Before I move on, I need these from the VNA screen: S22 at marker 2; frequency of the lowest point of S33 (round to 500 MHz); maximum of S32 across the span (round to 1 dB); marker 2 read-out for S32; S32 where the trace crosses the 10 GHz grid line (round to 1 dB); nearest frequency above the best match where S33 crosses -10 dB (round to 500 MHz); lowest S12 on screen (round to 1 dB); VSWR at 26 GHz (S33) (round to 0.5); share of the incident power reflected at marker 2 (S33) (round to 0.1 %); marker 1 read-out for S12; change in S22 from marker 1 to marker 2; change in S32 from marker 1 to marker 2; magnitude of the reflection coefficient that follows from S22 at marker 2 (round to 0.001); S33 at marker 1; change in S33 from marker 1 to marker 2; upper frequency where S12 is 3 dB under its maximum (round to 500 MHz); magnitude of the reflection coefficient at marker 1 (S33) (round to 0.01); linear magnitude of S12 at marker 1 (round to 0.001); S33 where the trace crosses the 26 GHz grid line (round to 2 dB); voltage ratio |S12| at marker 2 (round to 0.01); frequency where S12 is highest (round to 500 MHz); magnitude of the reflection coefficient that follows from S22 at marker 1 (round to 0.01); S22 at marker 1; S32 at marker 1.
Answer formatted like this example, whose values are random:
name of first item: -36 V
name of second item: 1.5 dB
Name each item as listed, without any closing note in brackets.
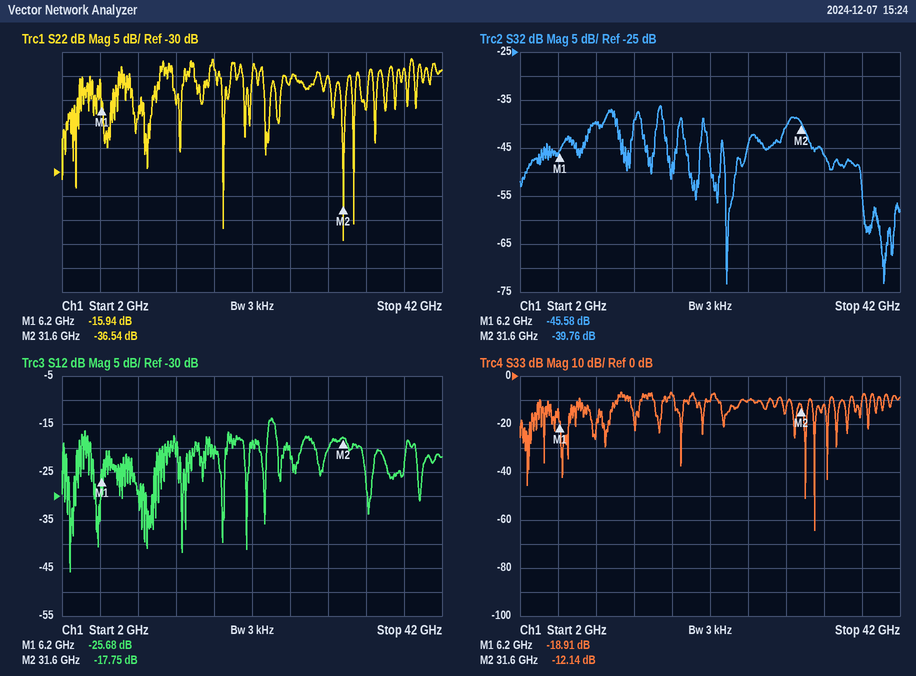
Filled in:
S22 at marker 2: -36.54 dB
frequency of the lowest point of S33: 33.0 GHz
maximum of S32 across the span: -36 dB
marker 2 read-out for S32: -39.76 dB
S32 where the trace crosses the 10 GHz grid line: -40 dB
nearest frequency above the best match where S33 crosses -10 dB: 34.5 GHz
lowest S12 on screen: -46 dB
VSWR at 26 GHz (S33): 2.0
share of the incident power reflected at marker 2 (S33): 6.1 %
marker 1 read-out for S12: -25.68 dB
change in S22 from marker 1 to marker 2: -20.60 dB
change in S32 from marker 1 to marker 2: 5.82 dB
magnitude of the reflection coefficient that follows from S22 at marker 2: 0.015
S33 at marker 1: -18.91 dB
change in S33 from marker 1 to marker 2: 6.77 dB
upper frequency where S12 is 3 dB under its maximum: 24.5 GHz
magnitude of the reflection coefficient at marker 1 (S33): 0.11
linear magnitude of S12 at marker 1: 0.052
S33 where the trace crosses the 26 GHz grid line: -10 dB
voltage ratio |S12| at marker 2: 0.13
frequency where S12 is highest: 24.0 GHz
magnitude of the reflection coefficient that follows from S22 at marker 1: 0.16
S22 at marker 1: -15.94 dB
S32 at marker 1: -45.58 dB
